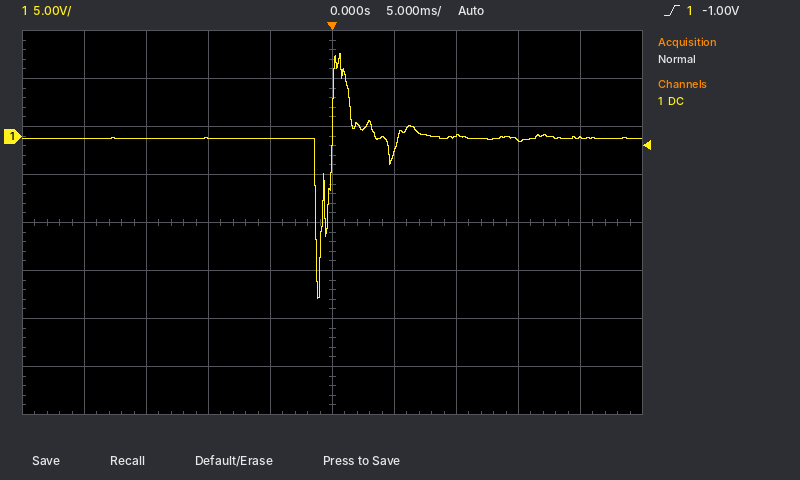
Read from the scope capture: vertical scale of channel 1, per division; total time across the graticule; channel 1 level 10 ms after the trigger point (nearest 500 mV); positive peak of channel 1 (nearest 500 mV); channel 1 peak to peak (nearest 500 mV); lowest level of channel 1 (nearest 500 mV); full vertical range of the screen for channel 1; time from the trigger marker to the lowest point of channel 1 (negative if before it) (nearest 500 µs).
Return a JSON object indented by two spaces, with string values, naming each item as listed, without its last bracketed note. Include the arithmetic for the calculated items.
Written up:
{
  "vertical scale of channel 1, per division": "5 V",
  "total time across the graticule": "50 ms",
  "channel 1 level 10 ms after the trigger point": "0.0 V",
  "positive peak of channel 1": "8.5 V",
  "channel 1 peak to peak": "8.5 V − (-17.0 V) = 25.5 V",
  "lowest level of channel 1": "-17.0 V",
  "full vertical range of the screen for channel 1": "40 V",
  "time from the trigger marker to the lowest point of channel 1 (negative if before it)": "-1.0 ms"
}
